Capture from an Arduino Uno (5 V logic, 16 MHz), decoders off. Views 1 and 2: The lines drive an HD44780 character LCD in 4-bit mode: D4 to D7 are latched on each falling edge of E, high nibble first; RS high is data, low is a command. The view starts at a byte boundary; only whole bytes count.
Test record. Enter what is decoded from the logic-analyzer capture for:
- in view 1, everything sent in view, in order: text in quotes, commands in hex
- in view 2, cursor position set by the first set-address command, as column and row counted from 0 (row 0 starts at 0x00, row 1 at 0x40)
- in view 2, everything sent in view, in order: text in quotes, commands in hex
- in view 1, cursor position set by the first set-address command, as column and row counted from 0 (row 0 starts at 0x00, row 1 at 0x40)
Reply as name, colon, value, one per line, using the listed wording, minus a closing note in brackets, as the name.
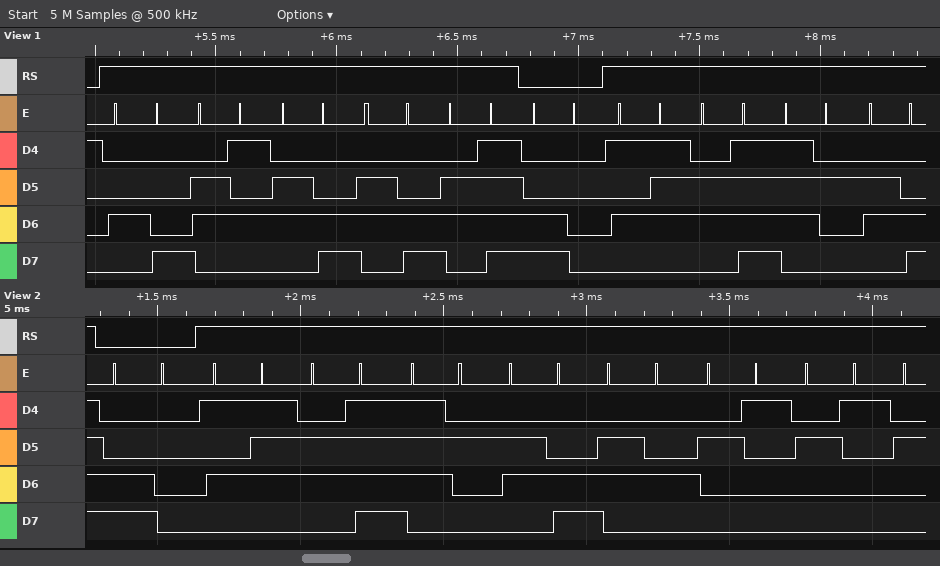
in view 1, everything sent in view, in order: text in quotes, commands in hex: "Hello" 0xC0 "Worl"
in view 2, cursor position set by the first set-address command, as column and row counted from 0: column 0, row 1
in view 2, everything sent in view, in order: text in quotes, commands in hex: 0xC0 "World!!"
in view 1, cursor position set by the first set-address command, as column and row counted from 0: column 0, row 1
